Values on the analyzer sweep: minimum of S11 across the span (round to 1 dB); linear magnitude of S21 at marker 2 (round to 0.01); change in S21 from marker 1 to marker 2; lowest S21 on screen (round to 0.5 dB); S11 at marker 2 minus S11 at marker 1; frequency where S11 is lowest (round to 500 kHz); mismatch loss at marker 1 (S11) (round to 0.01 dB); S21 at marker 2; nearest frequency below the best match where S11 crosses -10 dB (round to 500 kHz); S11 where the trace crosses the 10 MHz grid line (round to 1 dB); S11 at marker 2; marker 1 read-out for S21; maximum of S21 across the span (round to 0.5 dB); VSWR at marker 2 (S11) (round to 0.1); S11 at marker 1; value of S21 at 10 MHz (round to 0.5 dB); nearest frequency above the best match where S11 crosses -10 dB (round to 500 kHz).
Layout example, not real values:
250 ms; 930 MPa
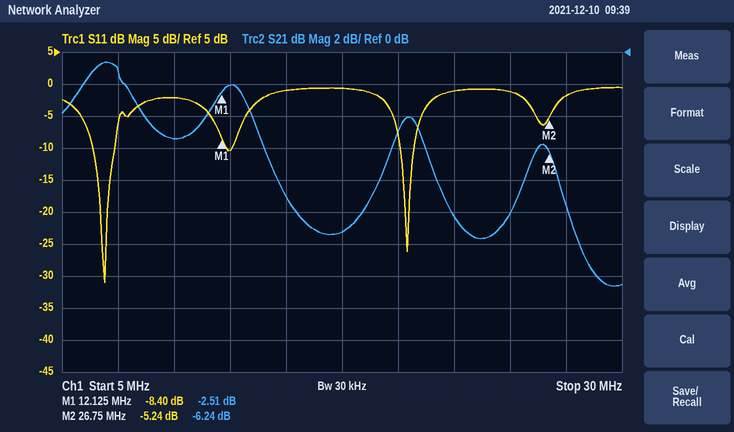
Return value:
-31 dB; 0.49; -3.73 dB; -14.5 dB; 3.16 dB; 7.0 MHz; 0.68 dB; -6.24 dB; 6.5 MHz; -2 dB; -5.24 dB; -2.51 dB; -0.5 dB; 3.4; -8.40 dB; -5.5 dB; 7.5 MHz
